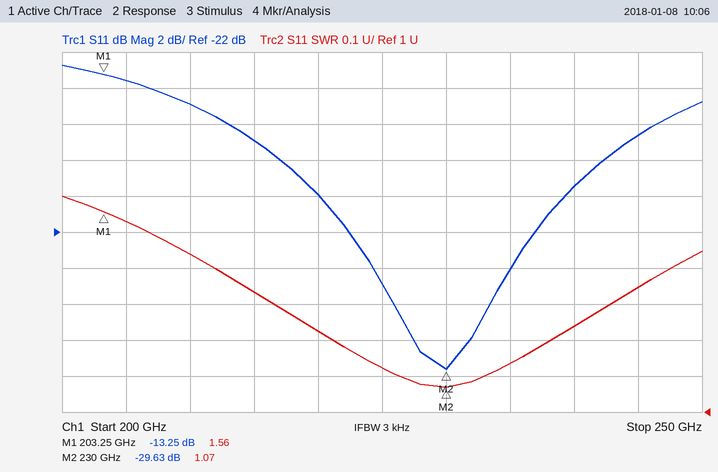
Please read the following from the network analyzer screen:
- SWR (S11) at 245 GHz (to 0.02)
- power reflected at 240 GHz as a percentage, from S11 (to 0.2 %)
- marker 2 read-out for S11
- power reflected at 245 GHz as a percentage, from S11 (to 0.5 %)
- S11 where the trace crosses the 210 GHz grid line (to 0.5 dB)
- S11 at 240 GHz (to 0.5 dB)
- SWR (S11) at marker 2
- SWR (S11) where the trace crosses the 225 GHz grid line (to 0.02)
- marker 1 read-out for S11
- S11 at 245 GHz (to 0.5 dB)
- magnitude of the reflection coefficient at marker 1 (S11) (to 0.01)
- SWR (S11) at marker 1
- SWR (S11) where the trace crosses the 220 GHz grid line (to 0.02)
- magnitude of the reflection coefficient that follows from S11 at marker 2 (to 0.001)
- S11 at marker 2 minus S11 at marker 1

1.34
1.2 %
-29.63 dB
2.0 %
-15.0 dB
-19.5 dB
1.07
1.12
-13.25 dB
-16.5 dB
0.22
1.56
1.22
0.033
-16.38 dB
